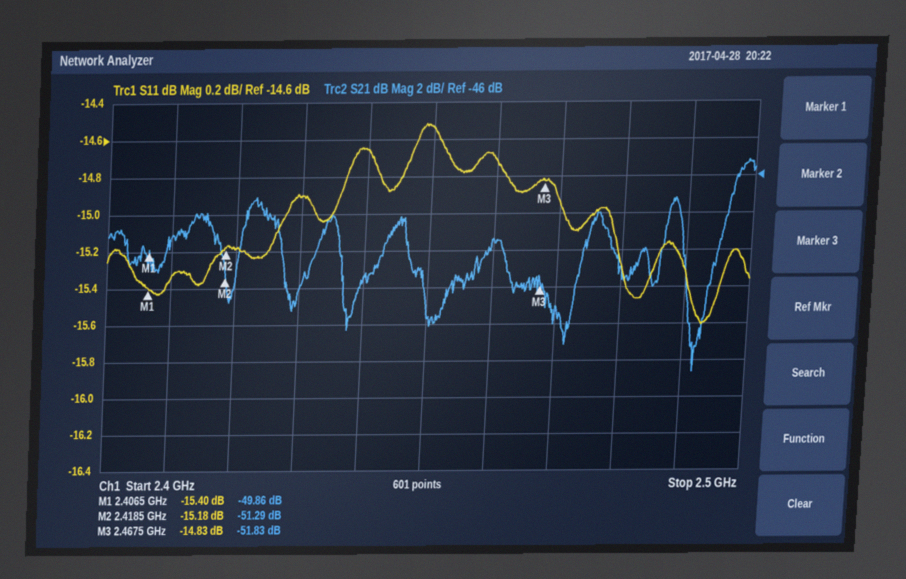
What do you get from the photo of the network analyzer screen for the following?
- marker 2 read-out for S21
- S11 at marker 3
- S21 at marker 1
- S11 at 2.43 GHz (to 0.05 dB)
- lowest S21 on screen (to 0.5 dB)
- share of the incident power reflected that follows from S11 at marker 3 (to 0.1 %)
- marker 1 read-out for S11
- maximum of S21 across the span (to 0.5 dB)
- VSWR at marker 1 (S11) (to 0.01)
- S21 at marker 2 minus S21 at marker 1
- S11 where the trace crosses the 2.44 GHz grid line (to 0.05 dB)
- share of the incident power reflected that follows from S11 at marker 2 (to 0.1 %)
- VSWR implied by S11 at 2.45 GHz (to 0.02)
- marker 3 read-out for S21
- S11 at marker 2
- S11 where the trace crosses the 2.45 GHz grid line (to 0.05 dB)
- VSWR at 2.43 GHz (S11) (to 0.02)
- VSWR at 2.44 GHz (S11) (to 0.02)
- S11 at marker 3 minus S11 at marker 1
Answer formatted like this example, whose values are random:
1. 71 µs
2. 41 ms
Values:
1. -51.29 dB
2. -14.83 dB
3. -49.86 dB
4. -14.90 dB
5. -56.5 dB
6. 3.3 %
7. -15.40 dB
8. -45.0 dB
9. 1.41
10. -1.43 dB
11. -14.65 dB
12. 3.0 %
13. 1.46
14. -51.83 dB
15. -15.18 dB
16. -14.55 dB
17. 1.44
18. 1.46
19. 0.57 dB
